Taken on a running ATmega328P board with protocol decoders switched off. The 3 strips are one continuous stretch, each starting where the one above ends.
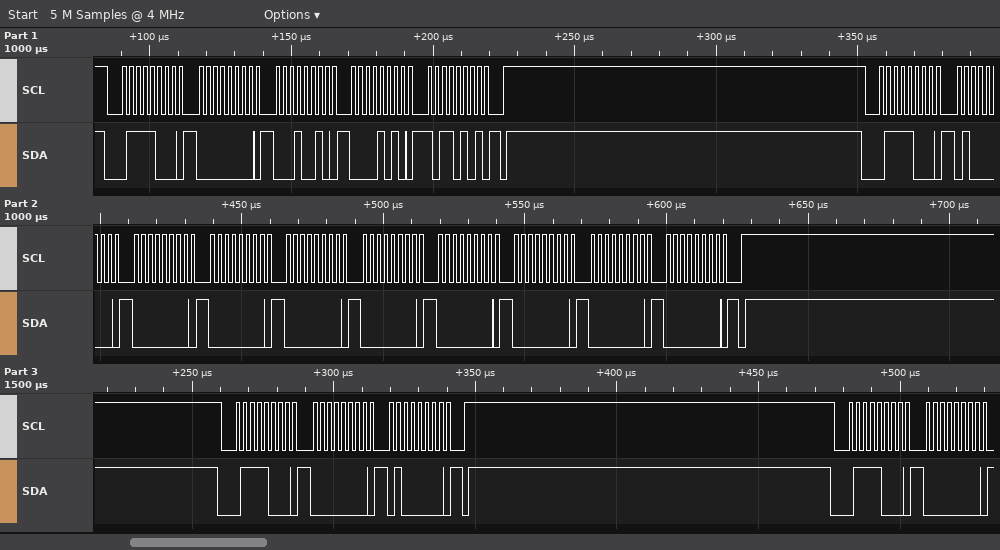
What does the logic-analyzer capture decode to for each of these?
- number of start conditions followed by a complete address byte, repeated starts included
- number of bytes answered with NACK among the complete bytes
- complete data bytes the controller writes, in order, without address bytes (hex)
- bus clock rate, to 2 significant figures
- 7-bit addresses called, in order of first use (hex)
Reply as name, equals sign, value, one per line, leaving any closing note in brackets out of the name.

number of start conditions followed by a complete address byte, repeated starts included = 4
number of bytes answered with NACK among the complete bytes = 0
complete data bytes the controller writes, in order, without address bytes = 00 12 0A B5 40 00 00 00 00 00 00 00 00 00 40 00
bus clock rate, to 2 significant figures = 400 kHz
7-bit addresses called, in order of first use = 0x3C
